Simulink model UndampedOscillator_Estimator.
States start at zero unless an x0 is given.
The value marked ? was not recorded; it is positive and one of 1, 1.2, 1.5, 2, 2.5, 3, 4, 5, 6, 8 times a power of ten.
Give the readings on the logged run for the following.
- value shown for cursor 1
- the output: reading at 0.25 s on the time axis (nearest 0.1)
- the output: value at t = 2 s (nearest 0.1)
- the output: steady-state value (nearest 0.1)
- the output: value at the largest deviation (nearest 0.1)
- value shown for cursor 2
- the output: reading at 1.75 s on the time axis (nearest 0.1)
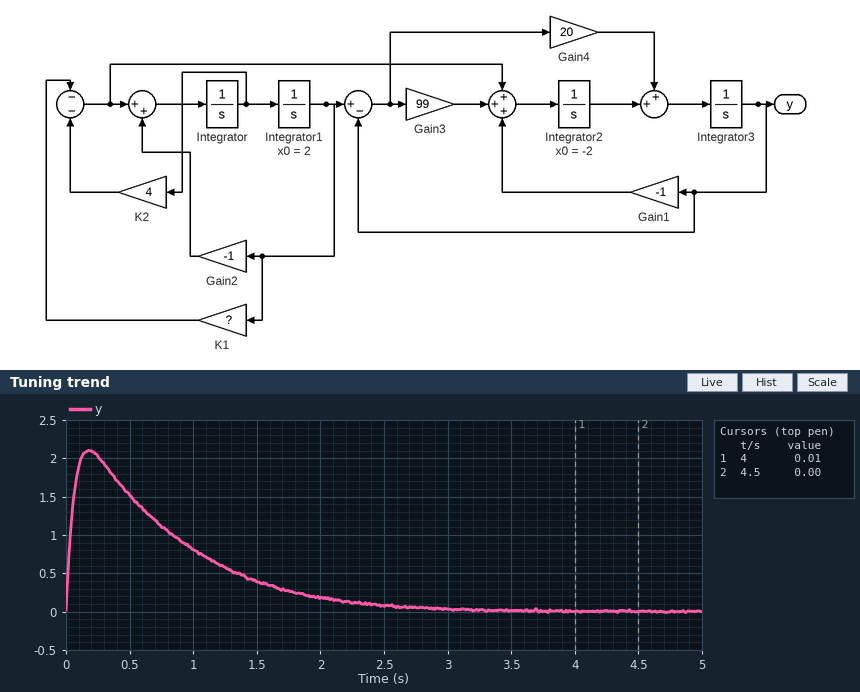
0.01
2.0
0.2
0.0
2.1
0.00
0.3
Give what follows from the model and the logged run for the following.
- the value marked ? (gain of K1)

3
